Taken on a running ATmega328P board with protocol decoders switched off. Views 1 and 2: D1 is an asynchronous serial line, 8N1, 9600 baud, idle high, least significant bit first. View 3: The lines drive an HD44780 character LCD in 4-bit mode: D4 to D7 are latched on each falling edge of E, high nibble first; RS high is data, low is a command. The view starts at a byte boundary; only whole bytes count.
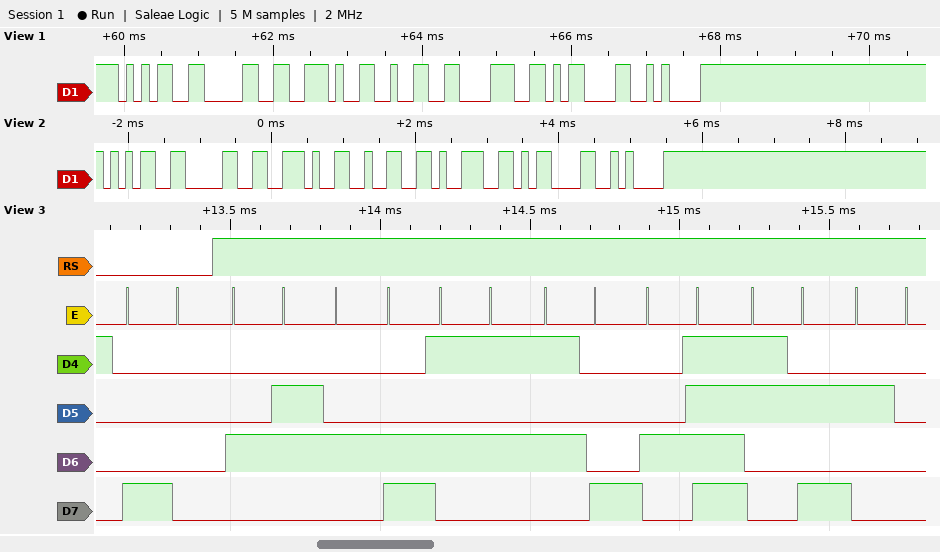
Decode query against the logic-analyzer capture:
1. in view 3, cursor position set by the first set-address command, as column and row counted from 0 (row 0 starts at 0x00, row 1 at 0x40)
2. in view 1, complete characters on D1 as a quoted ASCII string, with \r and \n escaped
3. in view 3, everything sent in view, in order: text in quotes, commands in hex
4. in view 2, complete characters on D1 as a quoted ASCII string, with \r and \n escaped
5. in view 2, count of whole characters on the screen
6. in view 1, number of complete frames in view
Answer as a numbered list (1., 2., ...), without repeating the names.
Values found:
1. column 0, row 0
2. "50.28\r\n"
3. 0x80 "FLUXO: "
4. "50.29\r\n"
5. 7
6. 7
